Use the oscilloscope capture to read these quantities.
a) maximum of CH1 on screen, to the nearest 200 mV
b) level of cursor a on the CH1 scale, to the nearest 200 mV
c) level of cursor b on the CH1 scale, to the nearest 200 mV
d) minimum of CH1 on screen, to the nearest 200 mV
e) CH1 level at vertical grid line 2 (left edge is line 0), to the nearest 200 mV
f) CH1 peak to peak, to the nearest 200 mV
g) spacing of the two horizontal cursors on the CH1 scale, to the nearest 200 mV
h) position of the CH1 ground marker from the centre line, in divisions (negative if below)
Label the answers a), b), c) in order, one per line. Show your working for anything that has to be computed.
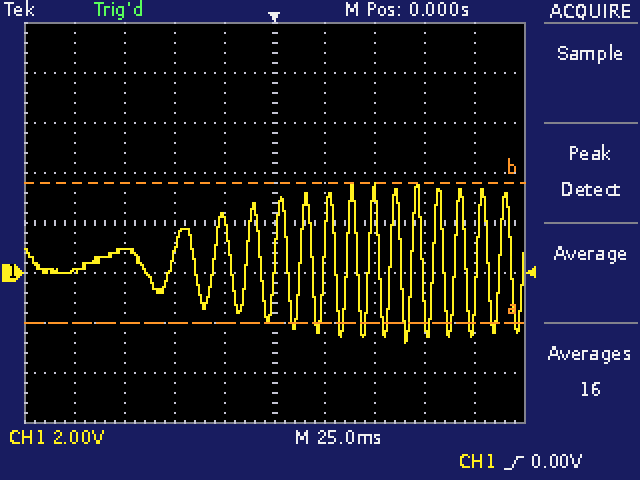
a) 3.6 V
b) -2.0 V
c) 3.6 V
d) -2.8 V
e) 1.0 V
f) 3.6 V − (-2.8 V) = 6.4 V
g) 5.6 V
h) -1.0 div
